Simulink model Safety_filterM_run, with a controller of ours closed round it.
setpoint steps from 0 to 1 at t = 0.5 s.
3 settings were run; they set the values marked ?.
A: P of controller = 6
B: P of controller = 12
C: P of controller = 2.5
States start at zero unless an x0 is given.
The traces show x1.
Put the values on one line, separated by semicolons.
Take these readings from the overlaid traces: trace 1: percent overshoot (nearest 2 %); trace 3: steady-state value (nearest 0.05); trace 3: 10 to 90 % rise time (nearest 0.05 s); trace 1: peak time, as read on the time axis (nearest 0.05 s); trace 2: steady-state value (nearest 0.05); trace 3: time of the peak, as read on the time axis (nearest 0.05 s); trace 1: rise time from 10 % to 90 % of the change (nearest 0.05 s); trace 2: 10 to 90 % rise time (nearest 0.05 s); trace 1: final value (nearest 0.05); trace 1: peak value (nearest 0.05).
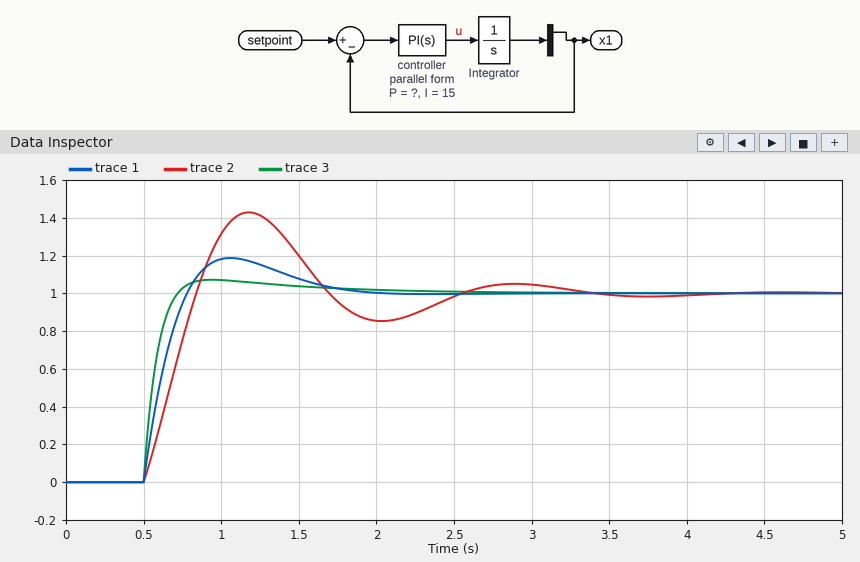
18 %; 1.00; 0.15 s; 1.05 s; 1.00; 0.95 s; 0.20 s; 0.25 s; 1.00; 1.20
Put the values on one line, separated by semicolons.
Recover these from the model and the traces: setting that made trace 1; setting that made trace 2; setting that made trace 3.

A; C; B
